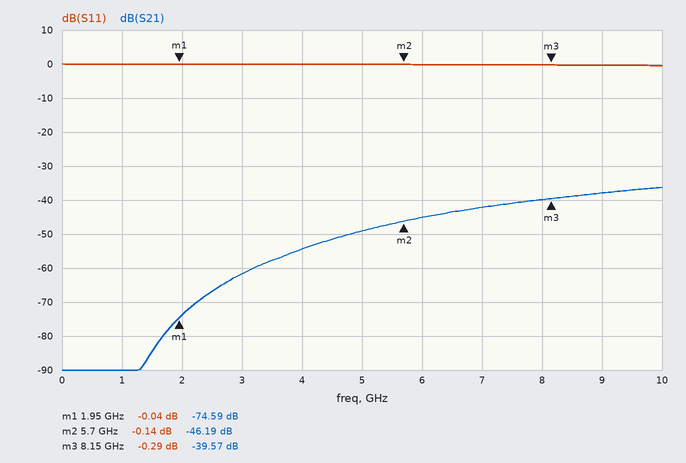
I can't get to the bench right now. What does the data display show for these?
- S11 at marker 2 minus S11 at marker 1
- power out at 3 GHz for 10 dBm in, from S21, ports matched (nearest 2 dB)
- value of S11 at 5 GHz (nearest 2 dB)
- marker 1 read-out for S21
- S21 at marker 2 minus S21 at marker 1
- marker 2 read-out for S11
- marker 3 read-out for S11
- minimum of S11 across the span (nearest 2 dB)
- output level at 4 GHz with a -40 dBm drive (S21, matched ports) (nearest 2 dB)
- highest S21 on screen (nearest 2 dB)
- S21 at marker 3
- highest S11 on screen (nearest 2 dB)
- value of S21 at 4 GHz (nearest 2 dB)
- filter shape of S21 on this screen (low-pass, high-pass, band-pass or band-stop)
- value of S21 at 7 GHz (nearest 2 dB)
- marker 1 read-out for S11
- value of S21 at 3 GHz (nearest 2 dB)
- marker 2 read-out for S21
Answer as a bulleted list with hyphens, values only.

- -0.10 dB
- -52 dBm
- 0 dB
- -74.59 dB
- 28.40 dB
- -0.14 dB
- -0.29 dB
- 0 dB
- -94 dBm
- -36 dB
- -39.57 dB
- 0 dB
- -54 dB
- high-pass
- -42 dB
- -0.04 dB
- -62 dB
- -46.19 dB
